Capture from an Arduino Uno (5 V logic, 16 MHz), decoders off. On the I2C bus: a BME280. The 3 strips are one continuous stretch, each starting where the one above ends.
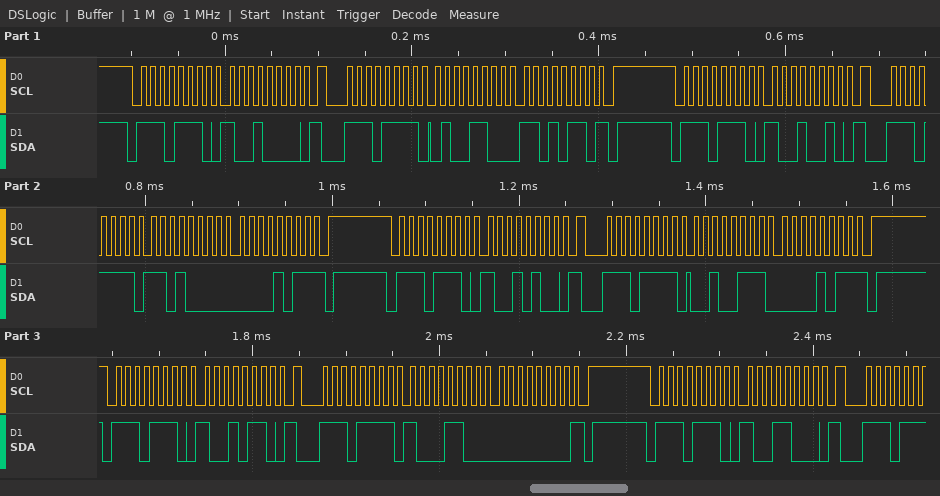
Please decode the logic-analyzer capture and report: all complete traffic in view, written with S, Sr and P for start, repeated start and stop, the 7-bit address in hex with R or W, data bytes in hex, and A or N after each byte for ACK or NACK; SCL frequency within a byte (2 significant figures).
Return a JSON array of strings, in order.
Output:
["S 77W A 90 A Sr 77R A 4C A D6 N P S 77W A 92 A Sr 77R A D0 A 0B N P S 77W A 94 A Sr 77R A 27 A 0B N P S 77W A 96 A Sr 77R A 8C A 00 N P S 77W A 98 A", "100 kHz"]
